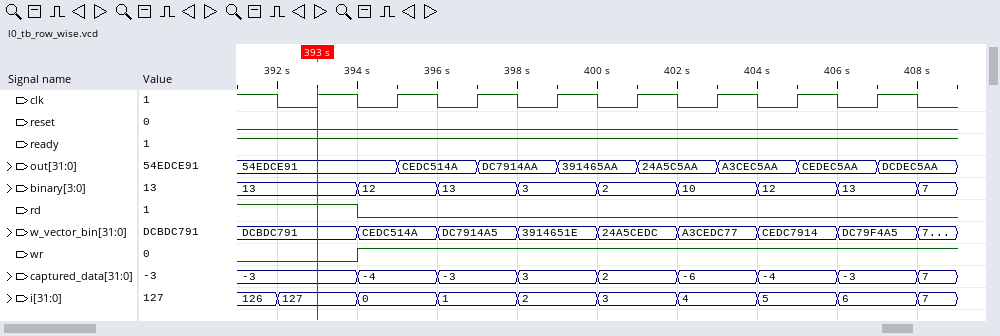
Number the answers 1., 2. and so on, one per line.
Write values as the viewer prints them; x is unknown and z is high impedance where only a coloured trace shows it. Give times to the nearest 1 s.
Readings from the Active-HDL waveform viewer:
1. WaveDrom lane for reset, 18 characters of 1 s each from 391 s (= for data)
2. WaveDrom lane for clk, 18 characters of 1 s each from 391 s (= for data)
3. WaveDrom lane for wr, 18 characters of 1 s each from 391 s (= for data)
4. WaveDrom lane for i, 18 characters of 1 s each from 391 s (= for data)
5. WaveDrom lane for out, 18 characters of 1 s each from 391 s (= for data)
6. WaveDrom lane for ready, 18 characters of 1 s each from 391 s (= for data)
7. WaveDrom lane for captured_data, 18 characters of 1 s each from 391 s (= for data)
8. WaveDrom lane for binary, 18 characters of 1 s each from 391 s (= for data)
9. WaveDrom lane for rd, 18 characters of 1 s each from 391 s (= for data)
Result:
1. {name: 'reset', wave: '0.................'}
2. {name: 'clk', wave: '101010101010101010'}
3. {name: 'wr', wave: '0..1..............'}
4. {name: 'i', wave: '==.=.=.=.=.=.=.=.=', data: '126 127 0 1 2 3 4 5 6 7'}
5. {name: 'out', wave: '=...=.=.=.=.=.=.=.', data: '54EDCE91 CEDC514A DC7914AA 391465AA 24A5C5AA A3CEC5AA CEDEC5AA DCDEC5AA'}
6. {name: 'ready', wave: '1.................'}
7. {name: 'captured_data', wave: '=..=.=.=.=.=.=.=.=', data: '-3 -4 -3 3 2 -6 -4 -3 7'}
8. {name: 'binary', wave: '=..=.=.=.=.=.=.=.=', data: '13 12 13 3 2 10 12 13 7'}
9. {name: 'rd', wave: '1..0..............'}
